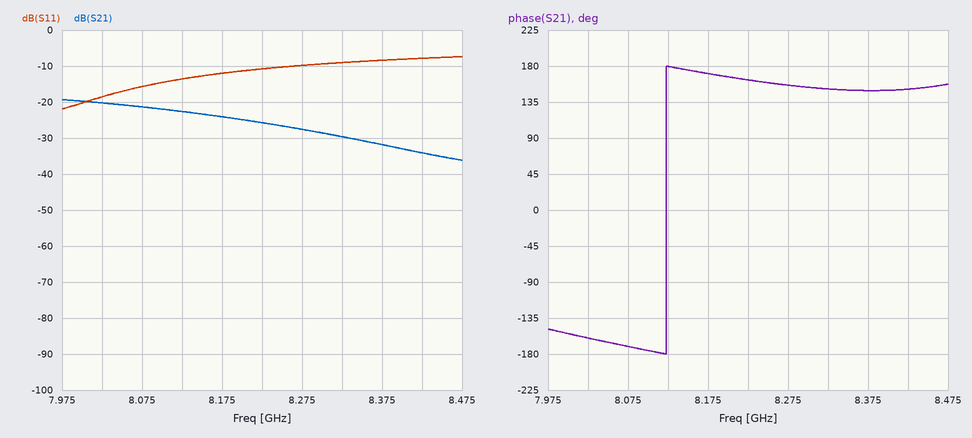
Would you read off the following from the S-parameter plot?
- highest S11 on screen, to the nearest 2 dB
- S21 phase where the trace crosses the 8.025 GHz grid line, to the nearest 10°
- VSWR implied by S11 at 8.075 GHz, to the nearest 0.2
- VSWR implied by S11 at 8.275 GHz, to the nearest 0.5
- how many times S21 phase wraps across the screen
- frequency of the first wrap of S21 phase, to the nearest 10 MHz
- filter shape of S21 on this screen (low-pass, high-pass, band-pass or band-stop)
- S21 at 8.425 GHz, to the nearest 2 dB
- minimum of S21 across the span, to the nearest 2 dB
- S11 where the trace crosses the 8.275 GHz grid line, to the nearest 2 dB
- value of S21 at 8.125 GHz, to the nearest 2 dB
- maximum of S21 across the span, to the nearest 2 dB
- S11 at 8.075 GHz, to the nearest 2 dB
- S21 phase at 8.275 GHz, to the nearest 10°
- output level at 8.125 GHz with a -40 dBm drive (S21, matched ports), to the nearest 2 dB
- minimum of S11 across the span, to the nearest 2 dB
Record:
-8 dB
-160°
1.4
2.0
1
8.12 GHz
low-pass
-34 dB
-36 dB
-10 dB
-22 dB
-20 dB
-16 dB
160°
-62 dBm
-22 dB
